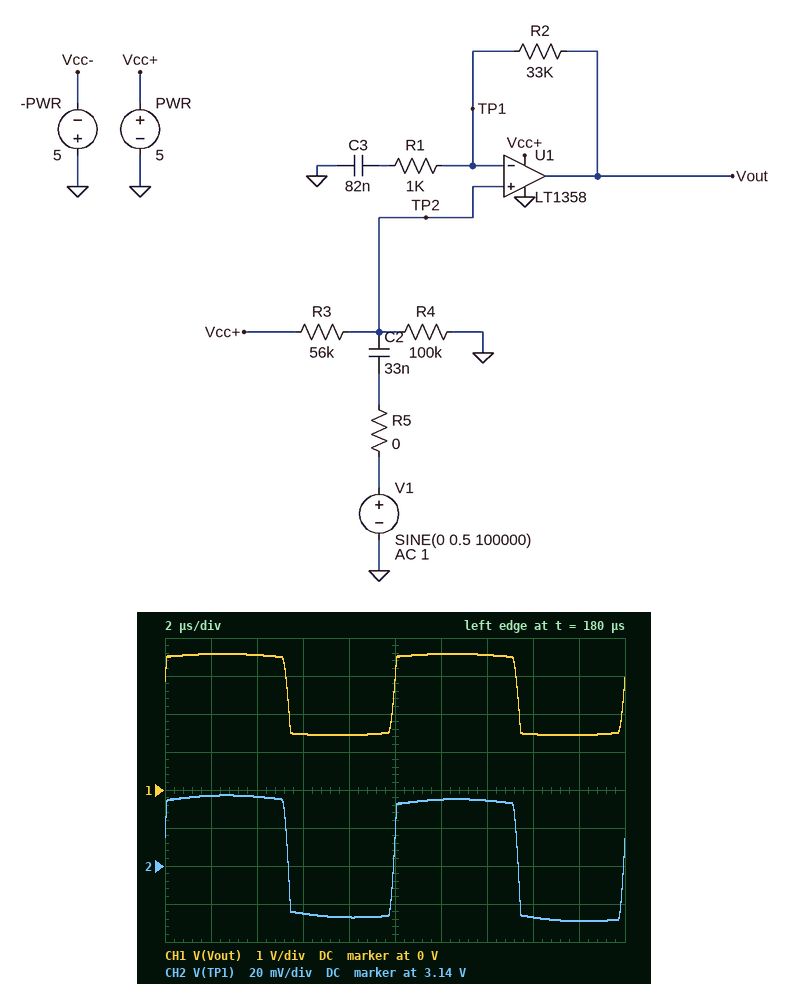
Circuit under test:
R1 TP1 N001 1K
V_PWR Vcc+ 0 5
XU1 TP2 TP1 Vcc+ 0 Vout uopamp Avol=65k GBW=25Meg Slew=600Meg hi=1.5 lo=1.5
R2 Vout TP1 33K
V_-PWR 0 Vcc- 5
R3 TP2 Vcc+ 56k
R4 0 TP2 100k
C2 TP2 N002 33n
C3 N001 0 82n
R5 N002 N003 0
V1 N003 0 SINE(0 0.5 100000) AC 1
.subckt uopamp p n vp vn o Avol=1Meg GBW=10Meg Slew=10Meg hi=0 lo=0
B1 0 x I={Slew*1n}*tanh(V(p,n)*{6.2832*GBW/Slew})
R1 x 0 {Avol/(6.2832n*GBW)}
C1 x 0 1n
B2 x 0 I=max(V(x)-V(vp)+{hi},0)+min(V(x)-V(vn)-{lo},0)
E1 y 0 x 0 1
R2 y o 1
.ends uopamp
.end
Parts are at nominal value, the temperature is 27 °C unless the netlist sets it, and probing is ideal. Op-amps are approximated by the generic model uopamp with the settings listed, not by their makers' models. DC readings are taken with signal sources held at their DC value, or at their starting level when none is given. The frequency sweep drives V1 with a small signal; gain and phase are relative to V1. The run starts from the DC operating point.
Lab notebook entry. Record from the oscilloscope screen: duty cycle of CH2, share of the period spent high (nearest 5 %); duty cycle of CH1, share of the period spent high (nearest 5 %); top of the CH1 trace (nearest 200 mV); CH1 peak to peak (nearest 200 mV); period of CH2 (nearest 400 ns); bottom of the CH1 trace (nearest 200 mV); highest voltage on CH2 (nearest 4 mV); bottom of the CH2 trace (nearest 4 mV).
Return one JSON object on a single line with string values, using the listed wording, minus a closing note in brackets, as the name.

{"duty cycle of CH2, share of the period spent high": "55 %", "duty cycle of CH1, share of the period spent high": "55 %", "top of the CH1 trace": "3.6 V", "CH1 peak to peak": "2.2 V", "period of CH2": "10.0 µs", "bottom of the CH1 trace": "1.4 V", "highest voltage on CH2": "3.176 V", "bottom of the CH2 trace": "3.112 V"}
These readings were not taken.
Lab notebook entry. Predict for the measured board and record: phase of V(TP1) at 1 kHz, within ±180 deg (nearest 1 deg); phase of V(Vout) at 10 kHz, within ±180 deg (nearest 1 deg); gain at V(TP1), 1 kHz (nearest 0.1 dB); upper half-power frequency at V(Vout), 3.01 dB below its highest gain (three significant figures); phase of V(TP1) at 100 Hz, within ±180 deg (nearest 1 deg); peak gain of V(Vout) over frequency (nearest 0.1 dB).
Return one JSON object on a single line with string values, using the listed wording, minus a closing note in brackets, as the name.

{"phase of V(TP1) at 1 kHz, within ±180 deg": "8 deg", "phase of V(Vout) at 10 kHz, within ±180 deg": "11 deg", "gain at V(TP1), 1 kHz": "-0.1 dB", "upper half-power frequency at V(Vout), 3.01 dB below its highest gain": "738 kHz", "phase of V(TP1) at 100 Hz, within ±180 deg": "53 deg", "peak gain of V(Vout) over frequency": "30.6 dB"}
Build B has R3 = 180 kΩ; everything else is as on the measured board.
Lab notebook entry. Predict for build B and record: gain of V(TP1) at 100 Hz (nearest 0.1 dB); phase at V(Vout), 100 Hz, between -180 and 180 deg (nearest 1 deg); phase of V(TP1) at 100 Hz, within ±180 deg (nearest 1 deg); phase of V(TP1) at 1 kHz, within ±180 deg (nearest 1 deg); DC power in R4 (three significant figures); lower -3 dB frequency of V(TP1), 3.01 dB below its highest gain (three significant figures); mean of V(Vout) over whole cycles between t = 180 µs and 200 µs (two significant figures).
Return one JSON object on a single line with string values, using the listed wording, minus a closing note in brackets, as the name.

{"gain of V(TP1) at 100 Hz": "-1.9 dB", "phase at V(Vout), 100 Hz, between -180 and 180 deg": "94 deg", "phase of V(TP1) at 100 Hz, within ±180 deg": "37 deg", "phase of V(TP1) at 1 kHz, within ±180 deg": "4 deg", "DC power in R4": "31.9 µW", "lower -3 dB frequency of V(TP1), 3.01 dB below its highest gain": "75.3 Hz", "mean of V(Vout) over whole cycles between t = 180 µs and 200 µs": "2.4 V"}
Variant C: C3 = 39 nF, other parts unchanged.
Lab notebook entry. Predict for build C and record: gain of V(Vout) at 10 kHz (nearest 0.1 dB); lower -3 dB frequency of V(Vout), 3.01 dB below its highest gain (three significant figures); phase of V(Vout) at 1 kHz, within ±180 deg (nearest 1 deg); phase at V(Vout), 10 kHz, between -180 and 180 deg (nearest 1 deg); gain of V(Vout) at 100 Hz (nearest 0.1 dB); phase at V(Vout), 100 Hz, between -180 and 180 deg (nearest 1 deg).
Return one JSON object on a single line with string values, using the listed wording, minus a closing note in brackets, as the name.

{"gain of V(Vout) at 10 kHz": "30.0 dB", "lower -3 dB frequency of V(Vout), 3.01 dB below its highest gain": "4.06 kHz", "phase of V(Vout) at 1 kHz, within ±180 deg": "77 deg", "phase at V(Vout), 10 kHz, between -180 and 180 deg": "22 deg", "gain of V(Vout) at 100 Hz": "-2.2 dB", "phase at V(Vout), 100 Hz, between -180 and 180 deg": "92 deg"}
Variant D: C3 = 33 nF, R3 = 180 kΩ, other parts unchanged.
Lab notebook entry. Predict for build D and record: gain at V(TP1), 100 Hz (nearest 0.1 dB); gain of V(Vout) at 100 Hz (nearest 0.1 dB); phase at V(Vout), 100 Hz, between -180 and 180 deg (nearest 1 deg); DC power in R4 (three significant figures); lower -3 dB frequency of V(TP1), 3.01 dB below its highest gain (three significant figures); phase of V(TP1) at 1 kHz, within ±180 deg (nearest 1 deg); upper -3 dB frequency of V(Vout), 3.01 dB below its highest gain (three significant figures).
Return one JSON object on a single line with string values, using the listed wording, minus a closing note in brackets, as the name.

{"gain at V(TP1), 100 Hz": "-1.9 dB", "gain of V(Vout) at 100 Hz": "-0.2 dB", "phase at V(Vout), 100 Hz, between -180 and 180 deg": "71 deg", "DC power in R4": "31.9 µW", "lower -3 dB frequency of V(TP1), 3.01 dB below its highest gain": "75.8 Hz", "phase of V(TP1) at 1 kHz, within ±180 deg": "4 deg", "upper -3 dB frequency of V(Vout), 3.01 dB below its highest gain": "741 kHz"}
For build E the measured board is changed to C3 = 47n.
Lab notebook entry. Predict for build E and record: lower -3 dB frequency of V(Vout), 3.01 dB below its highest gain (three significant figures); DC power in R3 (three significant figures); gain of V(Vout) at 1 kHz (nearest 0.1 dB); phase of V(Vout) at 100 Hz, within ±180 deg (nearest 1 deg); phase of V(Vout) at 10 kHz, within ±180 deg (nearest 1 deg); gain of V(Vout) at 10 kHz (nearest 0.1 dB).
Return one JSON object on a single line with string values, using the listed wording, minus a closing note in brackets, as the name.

{"lower -3 dB frequency of V(Vout), 3.01 dB below its highest gain": "3.37 kHz", "DC power in R3": "57.5 µW", "gain of V(Vout) at 1 kHz": "19.6 dB", "phase of V(Vout) at 100 Hz, within ±180 deg": "97 deg", "phase of V(Vout) at 10 kHz, within ±180 deg": "18 deg", "gain of V(Vout) at 10 kHz": "30.2 dB"}
